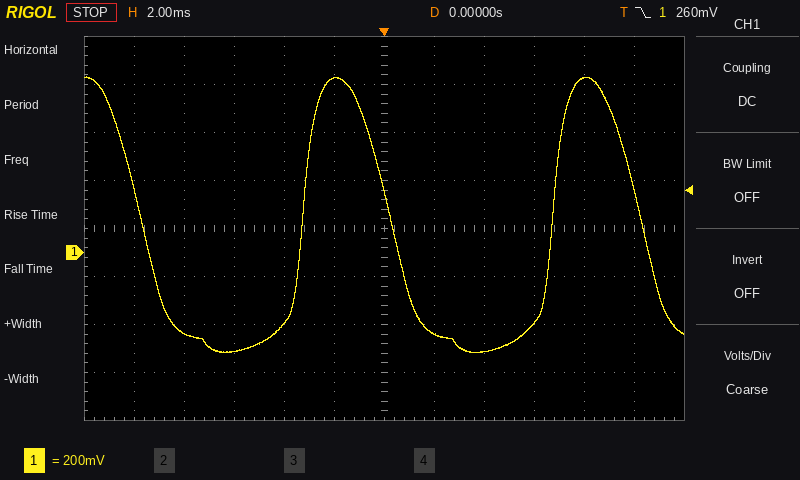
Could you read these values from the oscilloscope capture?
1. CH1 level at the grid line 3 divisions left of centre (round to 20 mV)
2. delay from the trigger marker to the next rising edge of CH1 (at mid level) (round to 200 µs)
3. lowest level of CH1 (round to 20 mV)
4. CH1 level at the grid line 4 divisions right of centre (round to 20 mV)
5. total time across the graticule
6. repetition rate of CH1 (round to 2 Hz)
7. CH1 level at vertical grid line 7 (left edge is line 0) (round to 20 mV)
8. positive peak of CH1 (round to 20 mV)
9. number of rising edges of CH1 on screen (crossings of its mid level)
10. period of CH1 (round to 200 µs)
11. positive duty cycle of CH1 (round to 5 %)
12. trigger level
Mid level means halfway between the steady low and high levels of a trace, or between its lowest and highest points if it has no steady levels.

-420 mV
6.8 ms
-420 mV
720 mV
24 ms
100 Hz
-340 mV
740 mV
2
10.0 ms
35 %
260 mV
